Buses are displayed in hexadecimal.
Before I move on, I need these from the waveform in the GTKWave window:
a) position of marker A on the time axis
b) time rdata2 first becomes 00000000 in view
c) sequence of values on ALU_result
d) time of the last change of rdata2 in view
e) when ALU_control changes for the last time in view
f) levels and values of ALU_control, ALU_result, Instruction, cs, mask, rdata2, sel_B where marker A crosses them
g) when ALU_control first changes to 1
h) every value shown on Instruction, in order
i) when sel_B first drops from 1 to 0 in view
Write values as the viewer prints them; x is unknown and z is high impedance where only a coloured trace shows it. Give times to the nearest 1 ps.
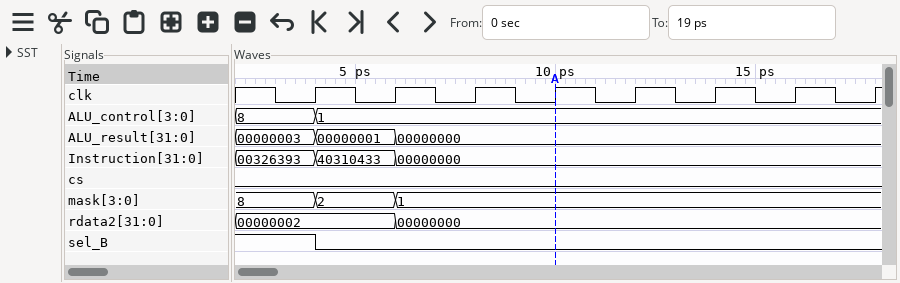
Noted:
10 ps
6 ps
00000003, 00000001, 00000000
6 ps
4 ps
ALU_control=1, ALU_result=00000000, Instruction=00000000, cs=0, mask=1, rdata2=00000000, sel_B=0
4 ps
00326393, 40310433, 00000000
4 ps
